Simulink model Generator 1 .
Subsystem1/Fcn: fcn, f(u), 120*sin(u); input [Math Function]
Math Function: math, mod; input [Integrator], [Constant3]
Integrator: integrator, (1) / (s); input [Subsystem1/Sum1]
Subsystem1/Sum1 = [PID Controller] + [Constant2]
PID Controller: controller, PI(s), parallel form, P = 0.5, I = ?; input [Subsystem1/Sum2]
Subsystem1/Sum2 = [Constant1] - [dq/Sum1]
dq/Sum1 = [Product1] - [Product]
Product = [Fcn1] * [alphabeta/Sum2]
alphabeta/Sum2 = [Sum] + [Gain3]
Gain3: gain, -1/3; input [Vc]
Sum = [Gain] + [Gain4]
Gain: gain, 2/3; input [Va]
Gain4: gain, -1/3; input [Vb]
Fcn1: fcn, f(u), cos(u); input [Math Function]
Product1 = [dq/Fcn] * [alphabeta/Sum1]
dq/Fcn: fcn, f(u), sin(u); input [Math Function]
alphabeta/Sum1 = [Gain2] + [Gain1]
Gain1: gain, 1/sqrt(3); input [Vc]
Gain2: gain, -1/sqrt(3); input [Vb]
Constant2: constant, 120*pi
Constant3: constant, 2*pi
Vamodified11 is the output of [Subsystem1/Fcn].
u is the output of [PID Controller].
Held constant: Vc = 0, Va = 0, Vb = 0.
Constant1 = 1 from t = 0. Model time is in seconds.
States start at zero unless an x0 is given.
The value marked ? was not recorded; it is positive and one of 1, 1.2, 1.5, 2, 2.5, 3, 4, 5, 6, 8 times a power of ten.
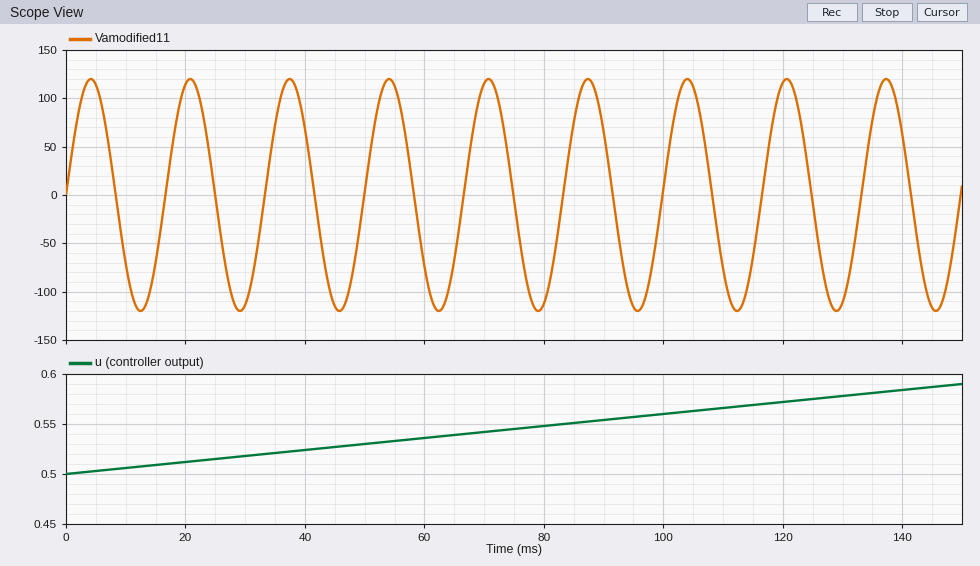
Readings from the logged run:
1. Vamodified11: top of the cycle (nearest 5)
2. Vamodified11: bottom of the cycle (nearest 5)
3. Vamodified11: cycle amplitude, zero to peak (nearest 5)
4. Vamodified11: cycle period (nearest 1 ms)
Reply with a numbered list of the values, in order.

1. 120
2. -120
3. 120
4. 17 ms
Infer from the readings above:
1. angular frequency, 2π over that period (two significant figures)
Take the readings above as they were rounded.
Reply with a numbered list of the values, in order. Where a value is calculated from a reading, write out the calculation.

1. 2π / 17 = 0.37 rad/ms
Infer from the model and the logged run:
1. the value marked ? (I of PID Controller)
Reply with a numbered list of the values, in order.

1. 0.6
